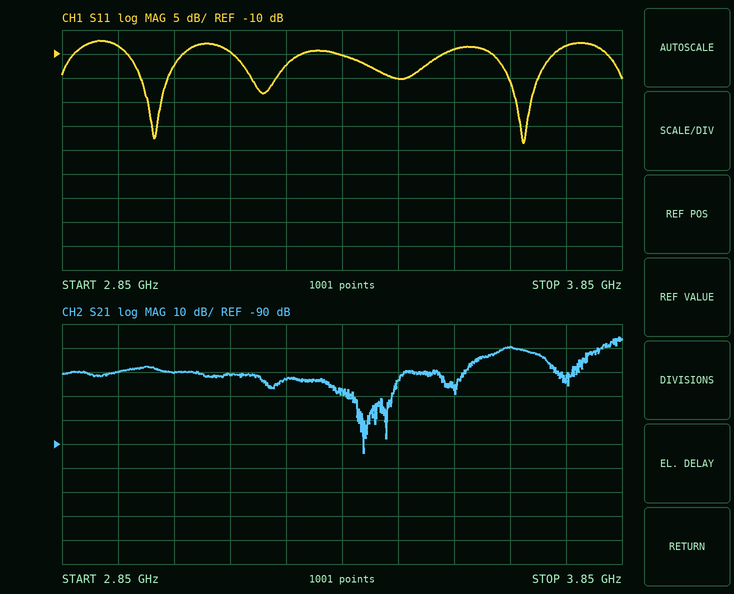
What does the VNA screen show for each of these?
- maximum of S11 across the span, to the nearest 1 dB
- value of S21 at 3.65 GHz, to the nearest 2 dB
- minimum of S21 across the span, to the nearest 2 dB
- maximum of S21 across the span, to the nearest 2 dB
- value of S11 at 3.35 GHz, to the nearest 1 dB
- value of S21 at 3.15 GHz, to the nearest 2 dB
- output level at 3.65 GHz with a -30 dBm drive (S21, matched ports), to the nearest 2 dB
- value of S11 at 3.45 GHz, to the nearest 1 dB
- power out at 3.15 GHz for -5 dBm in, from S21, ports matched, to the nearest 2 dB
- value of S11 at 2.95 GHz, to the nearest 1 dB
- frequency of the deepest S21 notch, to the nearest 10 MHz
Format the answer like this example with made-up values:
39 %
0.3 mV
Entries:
-7 dB
-50 dB
-94 dB
-46 dB
-10 dB
-62 dB
-80 dBm
-15 dB
-66 dBm
-8 dB
3.39 GHz
